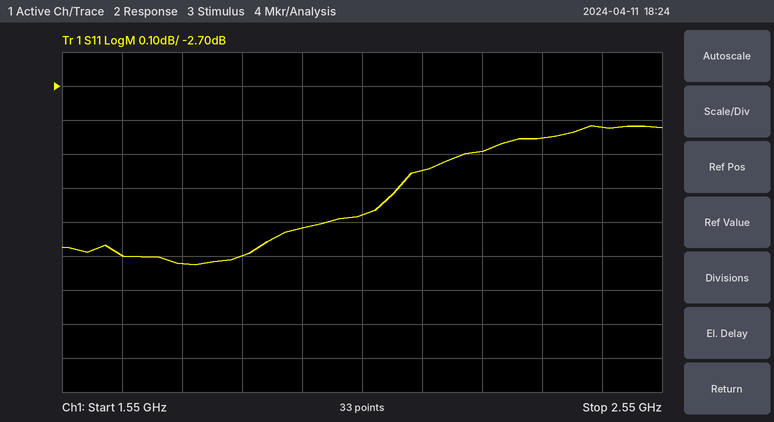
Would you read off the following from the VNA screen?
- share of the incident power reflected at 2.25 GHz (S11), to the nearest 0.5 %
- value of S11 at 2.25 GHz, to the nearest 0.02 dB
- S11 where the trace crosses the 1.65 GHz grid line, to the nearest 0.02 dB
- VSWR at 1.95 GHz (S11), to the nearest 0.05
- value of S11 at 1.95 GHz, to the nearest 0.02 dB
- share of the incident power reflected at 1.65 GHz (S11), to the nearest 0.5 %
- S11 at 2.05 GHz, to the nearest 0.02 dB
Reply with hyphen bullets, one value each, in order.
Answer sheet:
- 51.5 %
- -2.90 dB
- -3.20 dB
- 5.65
- -3.12 dB
- 48.0 %
- -3.08 dB
